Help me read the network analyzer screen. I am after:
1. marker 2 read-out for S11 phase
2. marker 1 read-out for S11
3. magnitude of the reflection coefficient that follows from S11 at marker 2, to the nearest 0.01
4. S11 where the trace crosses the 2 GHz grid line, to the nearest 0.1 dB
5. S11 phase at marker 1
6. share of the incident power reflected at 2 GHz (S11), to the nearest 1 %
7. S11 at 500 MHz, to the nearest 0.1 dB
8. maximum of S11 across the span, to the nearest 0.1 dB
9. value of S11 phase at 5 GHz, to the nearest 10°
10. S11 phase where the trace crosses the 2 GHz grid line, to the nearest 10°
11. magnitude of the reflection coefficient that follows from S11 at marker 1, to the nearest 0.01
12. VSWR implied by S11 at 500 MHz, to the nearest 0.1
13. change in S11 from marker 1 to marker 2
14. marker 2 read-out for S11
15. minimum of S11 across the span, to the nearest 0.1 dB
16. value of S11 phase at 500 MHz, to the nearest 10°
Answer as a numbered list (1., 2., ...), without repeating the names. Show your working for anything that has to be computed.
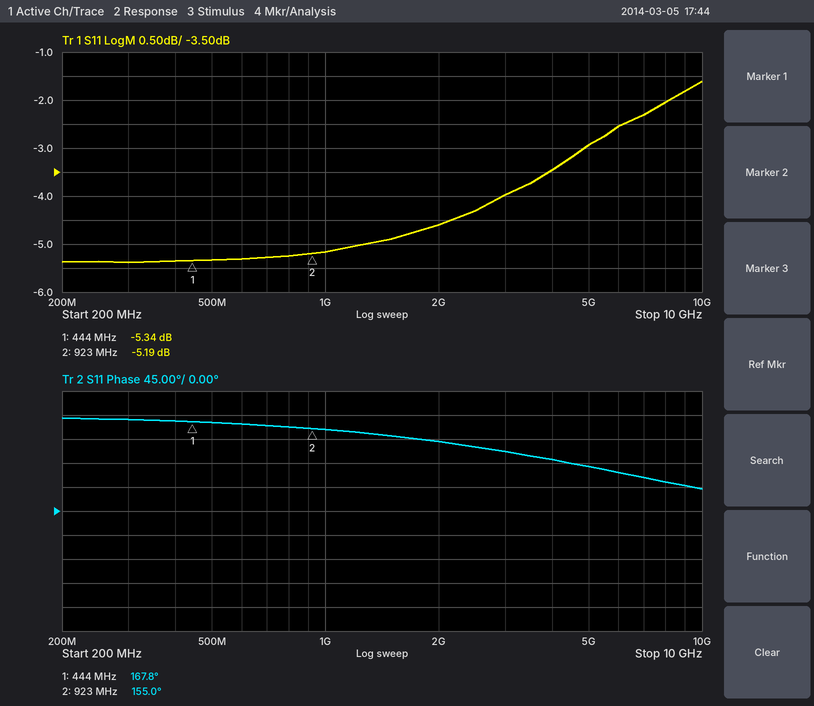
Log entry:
1. 155.0°
2. -5.34 dB
3. 10^(-5.19/20) ≈ 0.55
4. -4.6 dB
5. 167.8°
6. 10^(-4.6/10) ≈ 35 %
7. -5.3 dB
8. -1.6 dB
9. 80°
10. 130°
11. 10^(-5.34/20) ≈ 0.54
12. |Γ| = 10^(-5.3/20) = 0.5433; VSWR = (1 + 0.5433)/(1 − 0.5433) ≈ 3.4
13. -5.19 − (-5.34) = 0.15 dB
14. -5.19 dB
15. -5.4 dB
16. 170°
